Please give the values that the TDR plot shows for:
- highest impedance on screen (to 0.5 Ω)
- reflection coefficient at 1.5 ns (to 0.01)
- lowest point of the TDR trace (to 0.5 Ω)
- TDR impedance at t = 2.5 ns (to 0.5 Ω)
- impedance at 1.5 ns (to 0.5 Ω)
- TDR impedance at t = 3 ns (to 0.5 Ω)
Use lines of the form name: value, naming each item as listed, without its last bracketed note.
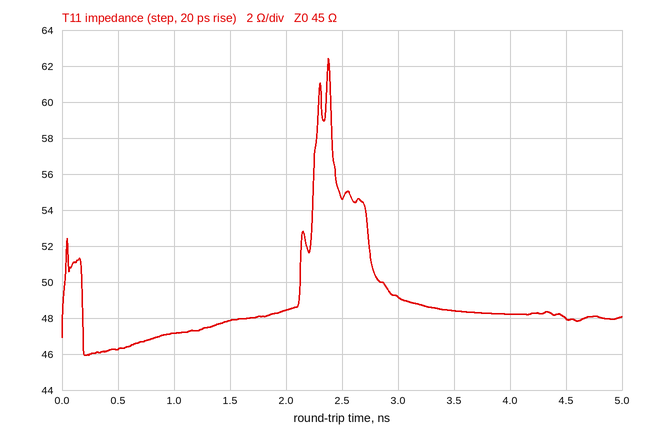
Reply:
highest impedance on screen: 62.5 Ω
reflection coefficient at 1.5 ns: +0.03
lowest point of the TDR trace: 46.0 Ω
TDR impedance at t = 2.5 ns: 54.5 Ω
impedance at 1.5 ns: 48.0 Ω
TDR impedance at t = 3 ns: 49.0 Ω
